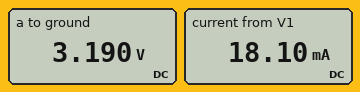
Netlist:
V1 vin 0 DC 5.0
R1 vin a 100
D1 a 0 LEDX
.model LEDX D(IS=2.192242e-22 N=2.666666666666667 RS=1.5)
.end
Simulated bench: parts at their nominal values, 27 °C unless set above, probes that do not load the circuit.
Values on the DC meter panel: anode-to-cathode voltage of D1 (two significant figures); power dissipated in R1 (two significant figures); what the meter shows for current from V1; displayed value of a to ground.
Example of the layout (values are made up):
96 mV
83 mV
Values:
3.2 V
33 mW
18.10 mA
3.190 V
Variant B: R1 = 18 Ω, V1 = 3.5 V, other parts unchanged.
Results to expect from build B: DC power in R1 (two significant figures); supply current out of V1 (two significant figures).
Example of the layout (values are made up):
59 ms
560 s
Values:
5.5 mW
17 mA
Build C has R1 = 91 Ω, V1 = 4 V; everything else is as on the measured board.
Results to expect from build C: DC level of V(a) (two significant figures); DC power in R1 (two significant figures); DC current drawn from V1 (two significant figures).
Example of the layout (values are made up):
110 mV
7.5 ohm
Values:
3.1 V
8.3 mW
9.5 mA
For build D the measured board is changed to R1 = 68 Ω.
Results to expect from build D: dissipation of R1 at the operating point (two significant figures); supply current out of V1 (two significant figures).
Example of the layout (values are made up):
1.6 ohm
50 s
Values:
46 mW
26 mA
